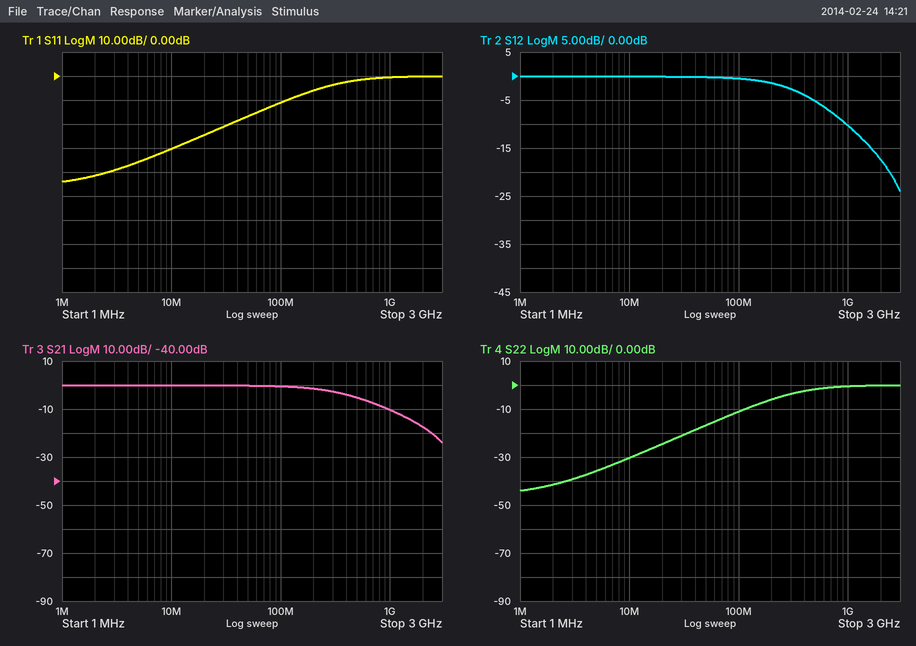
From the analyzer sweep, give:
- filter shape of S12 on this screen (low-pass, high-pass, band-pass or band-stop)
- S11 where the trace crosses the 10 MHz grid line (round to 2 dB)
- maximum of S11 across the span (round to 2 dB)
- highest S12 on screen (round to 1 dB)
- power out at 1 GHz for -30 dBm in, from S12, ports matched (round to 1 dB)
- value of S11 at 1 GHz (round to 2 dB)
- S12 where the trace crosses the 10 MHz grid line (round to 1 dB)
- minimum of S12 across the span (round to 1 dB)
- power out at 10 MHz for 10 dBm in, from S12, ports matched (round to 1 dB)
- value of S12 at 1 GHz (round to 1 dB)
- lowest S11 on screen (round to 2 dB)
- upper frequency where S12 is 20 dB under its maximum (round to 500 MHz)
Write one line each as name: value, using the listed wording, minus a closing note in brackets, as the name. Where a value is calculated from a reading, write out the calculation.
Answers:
filter shape of S12 on this screen: low-pass
S11 where the trace crosses the 10 MHz grid line: -30 dB
maximum of S11 across the span: 0 dB
highest S12 on screen: 0 dB
power out at 1 GHz for -30 dBm in, from S12, ports matched: -30 dBm + (-10 dB) = -40 dBm
value of S11 at 1 GHz: 0 dB
S12 where the trace crosses the 10 MHz grid line: 0 dB
minimum of S12 across the span: -24 dB
power out at 10 MHz for 10 dBm in, from S12, ports matched: 10 dBm + (0 dB) = 10 dBm
value of S12 at 1 GHz: -10 dB
lowest S11 on screen: -44 dB
upper frequency where S12 is 20 dB under its maximum: 2.5 GHz
